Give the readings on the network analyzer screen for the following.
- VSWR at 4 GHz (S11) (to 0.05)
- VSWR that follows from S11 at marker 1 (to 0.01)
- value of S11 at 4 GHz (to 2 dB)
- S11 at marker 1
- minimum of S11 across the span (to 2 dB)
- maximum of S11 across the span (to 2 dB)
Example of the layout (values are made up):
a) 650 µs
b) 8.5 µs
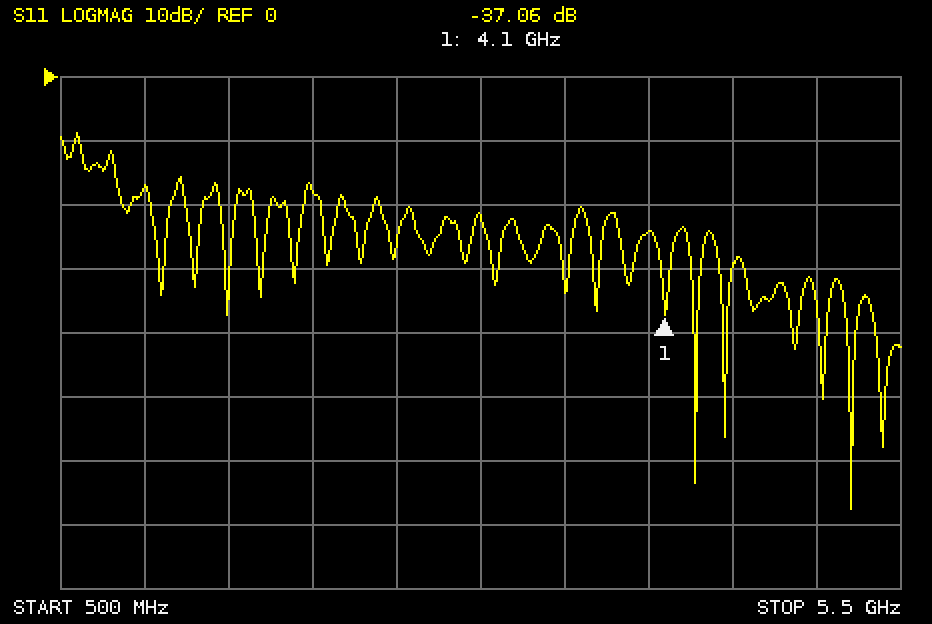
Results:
a) 1.15
b) 1.03
c) -24 dB
d) -37.06 dB
e) -68 dB
f) -8 dB
